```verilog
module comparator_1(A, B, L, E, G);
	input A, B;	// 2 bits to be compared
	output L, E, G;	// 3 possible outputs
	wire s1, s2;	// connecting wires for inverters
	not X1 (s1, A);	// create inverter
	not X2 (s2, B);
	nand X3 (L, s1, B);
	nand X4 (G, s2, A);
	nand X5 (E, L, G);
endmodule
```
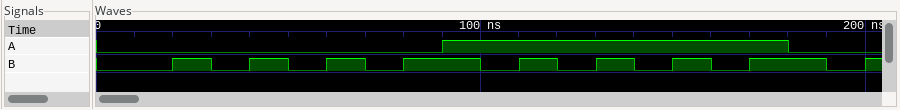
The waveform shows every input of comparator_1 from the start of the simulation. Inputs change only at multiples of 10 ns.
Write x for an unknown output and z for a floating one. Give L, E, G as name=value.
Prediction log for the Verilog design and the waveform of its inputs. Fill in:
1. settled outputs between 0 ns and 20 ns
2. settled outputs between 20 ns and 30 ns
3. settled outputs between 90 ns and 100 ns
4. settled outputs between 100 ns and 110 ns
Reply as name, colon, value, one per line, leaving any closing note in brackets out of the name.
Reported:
settled outputs between 0 ns and 20 ns: L=1, E=0, G=1
settled outputs between 20 ns and 30 ns: L=0, E=1, G=1
settled outputs between 90 ns and 100 ns: L=1, E=0, G=1
settled outputs between 100 ns and 110 ns: L=1, E=1, G=0
